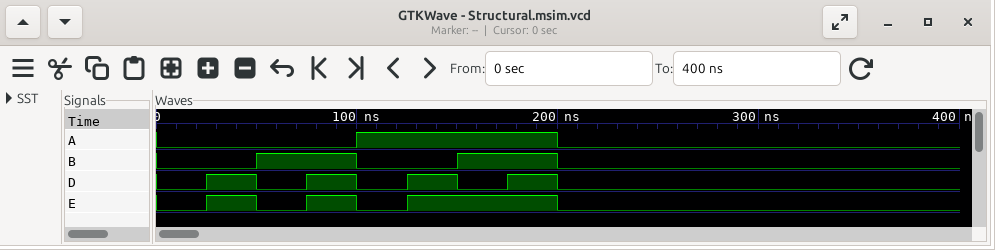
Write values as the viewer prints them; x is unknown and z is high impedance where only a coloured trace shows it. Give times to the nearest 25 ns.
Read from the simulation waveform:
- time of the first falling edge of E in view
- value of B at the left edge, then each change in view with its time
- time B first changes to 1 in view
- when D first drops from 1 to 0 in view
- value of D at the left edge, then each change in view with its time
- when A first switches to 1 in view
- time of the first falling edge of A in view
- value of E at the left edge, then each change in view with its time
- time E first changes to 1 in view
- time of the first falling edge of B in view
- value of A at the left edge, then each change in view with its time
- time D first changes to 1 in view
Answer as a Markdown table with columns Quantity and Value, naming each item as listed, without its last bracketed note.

| Quantity | Value |
|---|---|
| time of the first falling edge of E in view | 50 ns |
| value of B at the left edge, then each change in view with its time | 0, 1 at 50 ns, 0 at 100 ns, 1 at 150 ns, 0 at 200 ns |
| time B first changes to 1 in view | 50 ns |
| when D first drops from 1 to 0 in view | 50 ns |
| value of D at the left edge, then each change in view with its time | 0, 1 at 25 ns, 0 at 50 ns, 1 at 75 ns, 0 at 100 ns, 1 at 125 ns, 0 at 150 ns, 1 at 175 ns, 0 at 200 ns |
| when A first switches to 1 in view | 100 ns |
| time of the first falling edge of A in view | 200 ns |
| value of E at the left edge, then each change in view with its time | 0, 1 at 25 ns, 0 at 50 ns, 1 at 75 ns, 0 at 100 ns, 1 at 125 ns, 0 at 200 ns |
| time E first changes to 1 in view | 25 ns |
| time of the first falling edge of B in view | 100 ns |
| value of A at the left edge, then each change in view with its time | 0, 1 at 100 ns, 0 at 200 ns |
| time D first changes to 1 in view | 25 ns |
